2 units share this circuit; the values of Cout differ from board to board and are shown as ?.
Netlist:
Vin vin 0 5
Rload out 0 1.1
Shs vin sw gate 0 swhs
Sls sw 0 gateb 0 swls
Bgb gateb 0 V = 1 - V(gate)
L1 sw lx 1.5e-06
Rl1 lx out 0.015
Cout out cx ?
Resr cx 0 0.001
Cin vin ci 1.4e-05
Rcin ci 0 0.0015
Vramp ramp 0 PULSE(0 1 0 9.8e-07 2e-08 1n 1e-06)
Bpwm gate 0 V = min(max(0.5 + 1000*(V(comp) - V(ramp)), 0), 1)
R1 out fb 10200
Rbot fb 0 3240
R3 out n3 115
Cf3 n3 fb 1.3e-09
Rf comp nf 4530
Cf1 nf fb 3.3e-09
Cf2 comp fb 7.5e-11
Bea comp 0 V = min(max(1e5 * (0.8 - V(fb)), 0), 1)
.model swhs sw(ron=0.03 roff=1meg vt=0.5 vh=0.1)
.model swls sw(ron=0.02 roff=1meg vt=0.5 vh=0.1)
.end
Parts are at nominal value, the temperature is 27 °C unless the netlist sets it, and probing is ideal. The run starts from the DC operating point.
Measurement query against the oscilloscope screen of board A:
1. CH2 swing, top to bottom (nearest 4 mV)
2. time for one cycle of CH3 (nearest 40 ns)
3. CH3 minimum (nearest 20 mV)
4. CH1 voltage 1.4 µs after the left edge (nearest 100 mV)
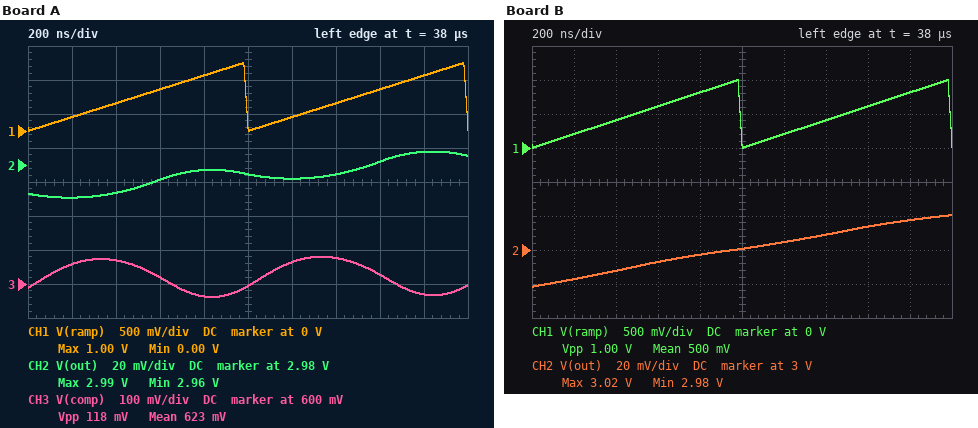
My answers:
28 mV
1.00 µs
560 mV
400 mV
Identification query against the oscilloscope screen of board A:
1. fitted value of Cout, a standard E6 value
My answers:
10 µF
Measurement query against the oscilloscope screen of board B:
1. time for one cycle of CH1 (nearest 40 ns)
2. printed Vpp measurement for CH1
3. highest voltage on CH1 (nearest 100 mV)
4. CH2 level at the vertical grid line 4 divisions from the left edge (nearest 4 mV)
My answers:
1.00 µs
1.00 V
1.0 V
2.996 V
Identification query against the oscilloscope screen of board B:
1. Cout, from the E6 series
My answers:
100 µF
